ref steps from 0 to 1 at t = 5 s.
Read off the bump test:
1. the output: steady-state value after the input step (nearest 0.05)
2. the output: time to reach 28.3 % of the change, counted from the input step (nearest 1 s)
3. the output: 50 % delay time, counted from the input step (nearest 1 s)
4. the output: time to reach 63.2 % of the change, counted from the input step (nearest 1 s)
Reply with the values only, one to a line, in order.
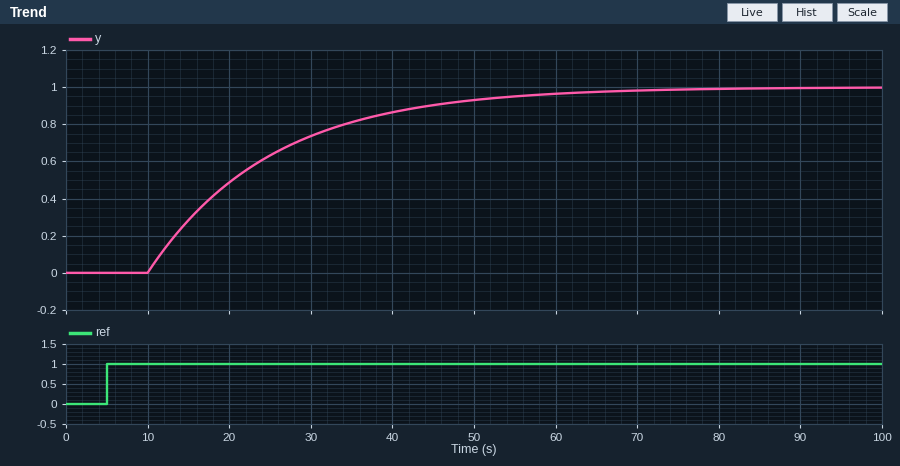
1.00
10 s
15 s
20 s
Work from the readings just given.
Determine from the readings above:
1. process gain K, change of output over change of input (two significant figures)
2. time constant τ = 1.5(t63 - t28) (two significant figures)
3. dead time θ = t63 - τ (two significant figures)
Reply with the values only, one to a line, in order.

1.0
15 s
5.0 s
